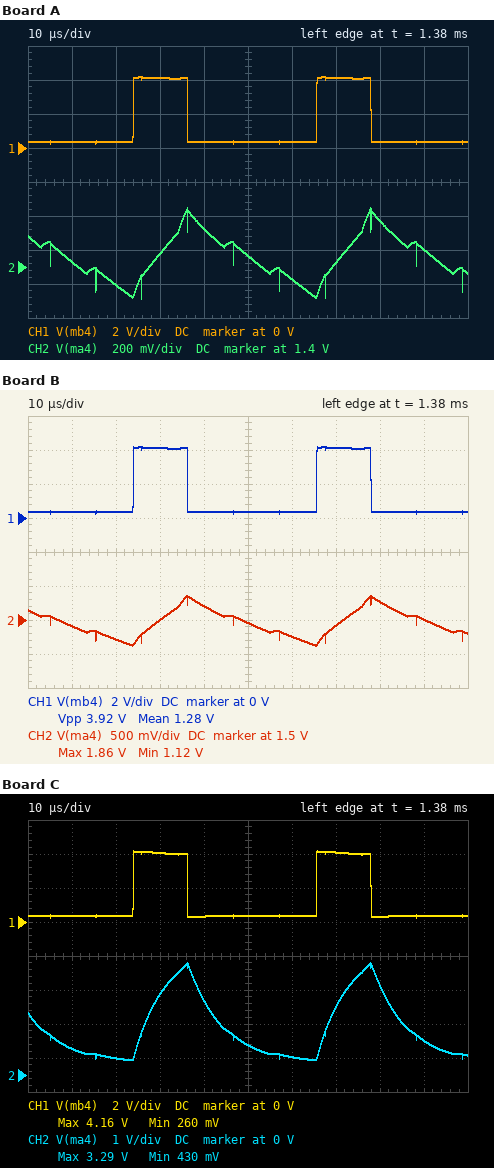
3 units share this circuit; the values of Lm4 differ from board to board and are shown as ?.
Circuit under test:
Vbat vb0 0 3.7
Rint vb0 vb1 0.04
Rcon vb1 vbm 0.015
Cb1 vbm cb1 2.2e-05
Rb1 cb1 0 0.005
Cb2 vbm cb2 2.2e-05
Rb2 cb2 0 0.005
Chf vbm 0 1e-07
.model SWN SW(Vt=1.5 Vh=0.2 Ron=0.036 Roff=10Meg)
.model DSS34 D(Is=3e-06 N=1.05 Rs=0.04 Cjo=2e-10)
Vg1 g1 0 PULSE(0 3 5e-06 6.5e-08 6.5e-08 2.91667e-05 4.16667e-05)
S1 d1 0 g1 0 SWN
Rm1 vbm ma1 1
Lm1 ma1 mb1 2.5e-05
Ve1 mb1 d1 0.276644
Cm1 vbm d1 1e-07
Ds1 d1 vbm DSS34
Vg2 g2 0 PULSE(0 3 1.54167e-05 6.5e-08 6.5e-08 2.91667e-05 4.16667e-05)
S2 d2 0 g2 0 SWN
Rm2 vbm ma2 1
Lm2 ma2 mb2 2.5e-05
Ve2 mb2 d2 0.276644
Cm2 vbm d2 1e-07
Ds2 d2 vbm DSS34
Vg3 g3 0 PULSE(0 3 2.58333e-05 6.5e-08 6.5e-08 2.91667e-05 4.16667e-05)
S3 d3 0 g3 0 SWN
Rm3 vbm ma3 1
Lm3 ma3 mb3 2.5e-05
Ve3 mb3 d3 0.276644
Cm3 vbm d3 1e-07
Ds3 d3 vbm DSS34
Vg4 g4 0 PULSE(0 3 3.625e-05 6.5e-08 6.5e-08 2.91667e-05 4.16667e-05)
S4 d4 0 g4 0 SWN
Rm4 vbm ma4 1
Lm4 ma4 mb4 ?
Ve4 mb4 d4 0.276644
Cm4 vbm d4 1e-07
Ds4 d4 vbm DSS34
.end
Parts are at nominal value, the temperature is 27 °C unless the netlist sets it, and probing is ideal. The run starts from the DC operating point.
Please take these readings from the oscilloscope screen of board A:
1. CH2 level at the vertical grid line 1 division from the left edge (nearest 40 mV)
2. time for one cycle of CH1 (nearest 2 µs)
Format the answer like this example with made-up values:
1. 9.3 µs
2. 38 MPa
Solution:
1. 1.44 V
2. 42 µs
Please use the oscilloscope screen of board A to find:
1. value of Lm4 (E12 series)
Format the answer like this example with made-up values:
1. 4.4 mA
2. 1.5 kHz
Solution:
1. 68 µH
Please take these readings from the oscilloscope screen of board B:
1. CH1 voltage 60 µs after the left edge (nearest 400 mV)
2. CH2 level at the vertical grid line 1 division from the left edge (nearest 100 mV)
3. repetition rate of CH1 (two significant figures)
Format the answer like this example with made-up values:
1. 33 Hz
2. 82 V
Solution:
1. 400 mV
2. 1.4 V
3. 24 kHz
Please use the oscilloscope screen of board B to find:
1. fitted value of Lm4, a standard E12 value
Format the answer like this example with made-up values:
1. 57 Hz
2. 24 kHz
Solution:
1. 47 µH
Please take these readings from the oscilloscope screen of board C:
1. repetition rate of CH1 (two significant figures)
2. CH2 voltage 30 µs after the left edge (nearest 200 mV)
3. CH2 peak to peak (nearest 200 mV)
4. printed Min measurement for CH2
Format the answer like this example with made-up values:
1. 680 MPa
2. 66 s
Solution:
1. 24 kHz
2. 2.4 V
3. 2.8 V
4. 430 mV
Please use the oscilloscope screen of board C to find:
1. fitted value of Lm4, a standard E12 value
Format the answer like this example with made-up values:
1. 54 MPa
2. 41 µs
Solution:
1. 8.2 µH
